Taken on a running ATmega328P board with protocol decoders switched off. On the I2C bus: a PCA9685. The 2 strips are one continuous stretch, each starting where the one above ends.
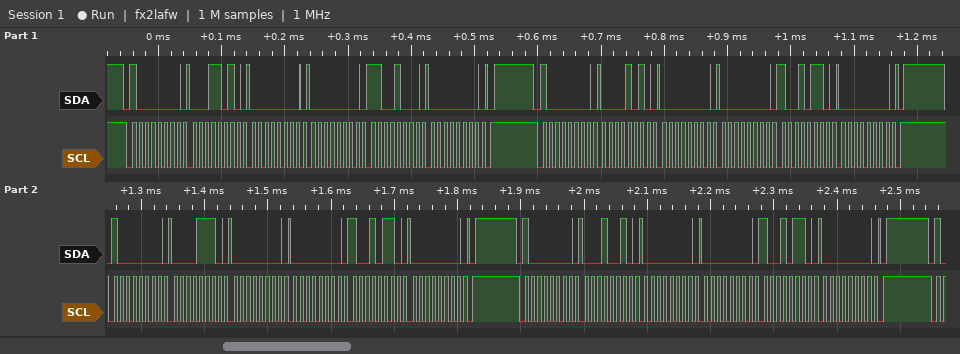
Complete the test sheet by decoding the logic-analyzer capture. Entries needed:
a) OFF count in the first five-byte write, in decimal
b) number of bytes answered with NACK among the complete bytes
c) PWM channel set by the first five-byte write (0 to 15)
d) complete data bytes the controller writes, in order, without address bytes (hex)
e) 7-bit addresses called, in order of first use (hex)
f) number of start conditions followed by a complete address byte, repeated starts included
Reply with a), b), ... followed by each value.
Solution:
a) 200
b) 0
c) 5
d) 1A 00 00 C8 00 0A 00 00 96 00 0E 00 00 96 00 12 00 00 96 00
e) 0x40
f) 4
